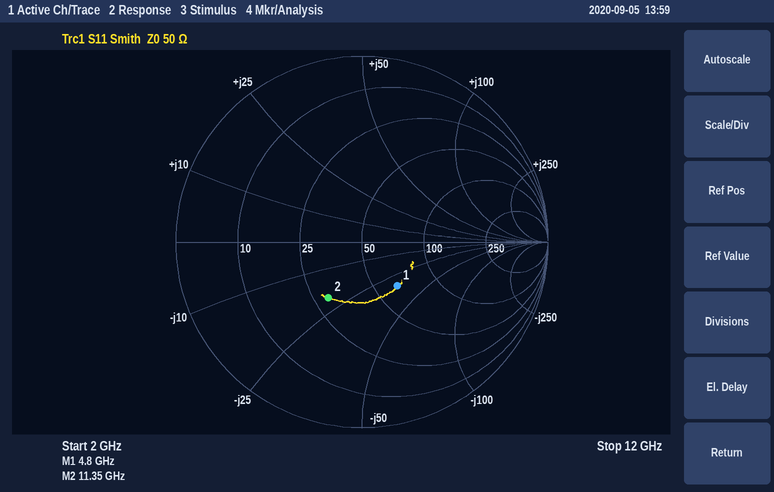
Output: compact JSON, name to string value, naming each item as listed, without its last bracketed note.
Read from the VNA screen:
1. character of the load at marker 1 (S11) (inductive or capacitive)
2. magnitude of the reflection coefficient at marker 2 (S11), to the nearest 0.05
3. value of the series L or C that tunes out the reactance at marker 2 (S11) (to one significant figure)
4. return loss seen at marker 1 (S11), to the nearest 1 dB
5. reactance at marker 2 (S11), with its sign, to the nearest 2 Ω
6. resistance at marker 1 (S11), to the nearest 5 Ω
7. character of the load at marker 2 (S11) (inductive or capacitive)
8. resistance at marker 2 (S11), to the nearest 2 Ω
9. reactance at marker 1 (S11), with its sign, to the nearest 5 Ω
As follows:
{"character of the load at marker 1 (S11)": "capacitive", "magnitude of the reflection coefficient at marker 2 (S11), to the nearest 0.05": "0.35", "value of the series L or C that tunes out the reactance at marker 2 (S11)": "300 pH", "return loss seen at marker 1 (S11), to the nearest 1 dB": "10 dB", "reactance at marker 2 (S11), with its sign, to the nearest 2 Ω": "-20 Ω", "resistance at marker 1 (S11), to the nearest 5 Ω": "65 Ω", "character of the load at marker 2 (S11)": "capacitive", "resistance at marker 2 (S11), to the nearest 2 Ω": "30 Ω", "reactance at marker 1 (S11), with its sign, to the nearest 5 Ω": "-35 Ω"}
